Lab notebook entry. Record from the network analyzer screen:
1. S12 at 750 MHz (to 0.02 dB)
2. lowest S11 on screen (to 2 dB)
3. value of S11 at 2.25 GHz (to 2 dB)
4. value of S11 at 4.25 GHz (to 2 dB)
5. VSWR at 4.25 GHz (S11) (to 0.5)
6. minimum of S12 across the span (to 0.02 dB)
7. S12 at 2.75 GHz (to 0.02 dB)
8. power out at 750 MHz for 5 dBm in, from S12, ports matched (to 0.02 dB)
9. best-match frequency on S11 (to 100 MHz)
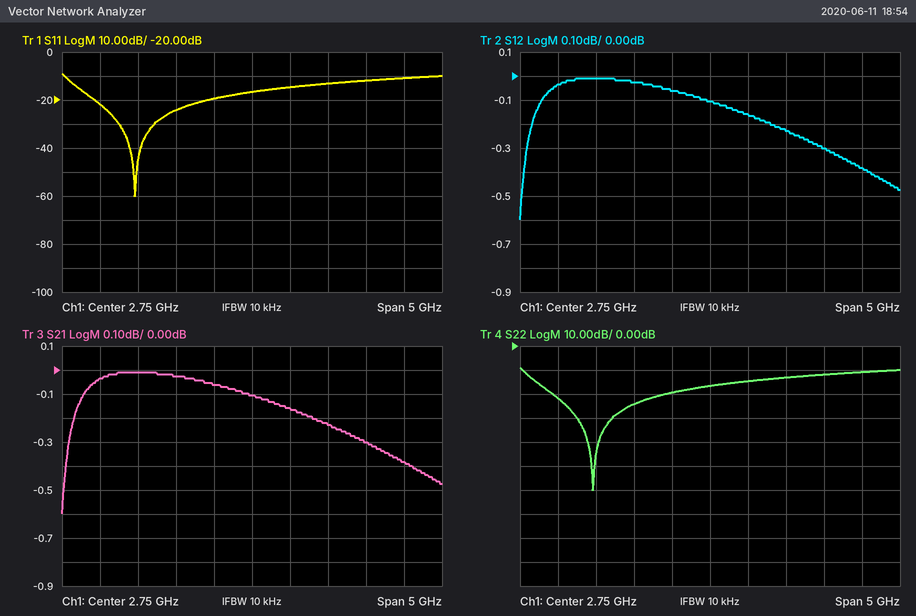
-0.04 dB
-60 dB
-20 dB
-12 dB
1.5
-0.60 dB
-0.10 dB
4.96 dBm
1.2 GHz
